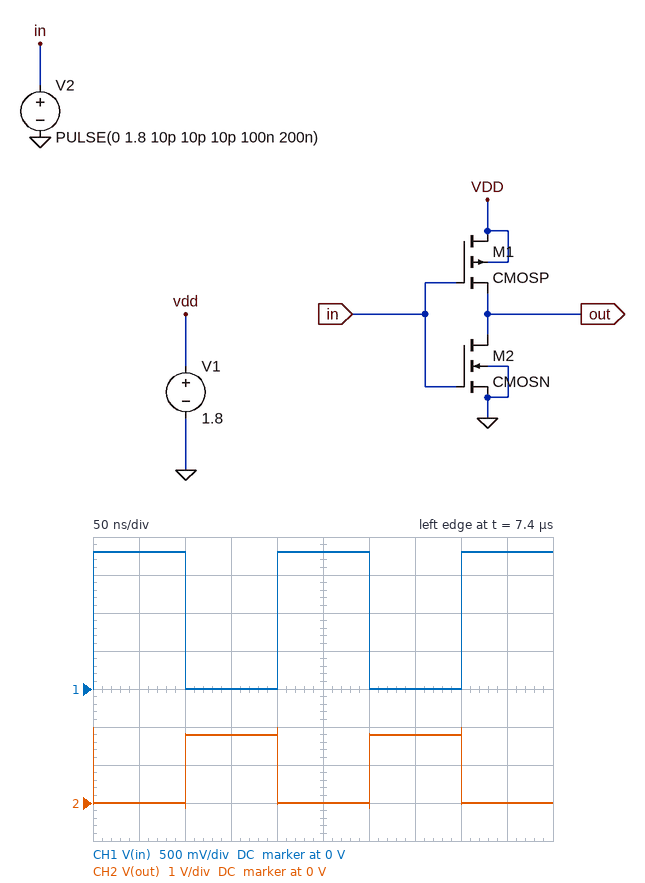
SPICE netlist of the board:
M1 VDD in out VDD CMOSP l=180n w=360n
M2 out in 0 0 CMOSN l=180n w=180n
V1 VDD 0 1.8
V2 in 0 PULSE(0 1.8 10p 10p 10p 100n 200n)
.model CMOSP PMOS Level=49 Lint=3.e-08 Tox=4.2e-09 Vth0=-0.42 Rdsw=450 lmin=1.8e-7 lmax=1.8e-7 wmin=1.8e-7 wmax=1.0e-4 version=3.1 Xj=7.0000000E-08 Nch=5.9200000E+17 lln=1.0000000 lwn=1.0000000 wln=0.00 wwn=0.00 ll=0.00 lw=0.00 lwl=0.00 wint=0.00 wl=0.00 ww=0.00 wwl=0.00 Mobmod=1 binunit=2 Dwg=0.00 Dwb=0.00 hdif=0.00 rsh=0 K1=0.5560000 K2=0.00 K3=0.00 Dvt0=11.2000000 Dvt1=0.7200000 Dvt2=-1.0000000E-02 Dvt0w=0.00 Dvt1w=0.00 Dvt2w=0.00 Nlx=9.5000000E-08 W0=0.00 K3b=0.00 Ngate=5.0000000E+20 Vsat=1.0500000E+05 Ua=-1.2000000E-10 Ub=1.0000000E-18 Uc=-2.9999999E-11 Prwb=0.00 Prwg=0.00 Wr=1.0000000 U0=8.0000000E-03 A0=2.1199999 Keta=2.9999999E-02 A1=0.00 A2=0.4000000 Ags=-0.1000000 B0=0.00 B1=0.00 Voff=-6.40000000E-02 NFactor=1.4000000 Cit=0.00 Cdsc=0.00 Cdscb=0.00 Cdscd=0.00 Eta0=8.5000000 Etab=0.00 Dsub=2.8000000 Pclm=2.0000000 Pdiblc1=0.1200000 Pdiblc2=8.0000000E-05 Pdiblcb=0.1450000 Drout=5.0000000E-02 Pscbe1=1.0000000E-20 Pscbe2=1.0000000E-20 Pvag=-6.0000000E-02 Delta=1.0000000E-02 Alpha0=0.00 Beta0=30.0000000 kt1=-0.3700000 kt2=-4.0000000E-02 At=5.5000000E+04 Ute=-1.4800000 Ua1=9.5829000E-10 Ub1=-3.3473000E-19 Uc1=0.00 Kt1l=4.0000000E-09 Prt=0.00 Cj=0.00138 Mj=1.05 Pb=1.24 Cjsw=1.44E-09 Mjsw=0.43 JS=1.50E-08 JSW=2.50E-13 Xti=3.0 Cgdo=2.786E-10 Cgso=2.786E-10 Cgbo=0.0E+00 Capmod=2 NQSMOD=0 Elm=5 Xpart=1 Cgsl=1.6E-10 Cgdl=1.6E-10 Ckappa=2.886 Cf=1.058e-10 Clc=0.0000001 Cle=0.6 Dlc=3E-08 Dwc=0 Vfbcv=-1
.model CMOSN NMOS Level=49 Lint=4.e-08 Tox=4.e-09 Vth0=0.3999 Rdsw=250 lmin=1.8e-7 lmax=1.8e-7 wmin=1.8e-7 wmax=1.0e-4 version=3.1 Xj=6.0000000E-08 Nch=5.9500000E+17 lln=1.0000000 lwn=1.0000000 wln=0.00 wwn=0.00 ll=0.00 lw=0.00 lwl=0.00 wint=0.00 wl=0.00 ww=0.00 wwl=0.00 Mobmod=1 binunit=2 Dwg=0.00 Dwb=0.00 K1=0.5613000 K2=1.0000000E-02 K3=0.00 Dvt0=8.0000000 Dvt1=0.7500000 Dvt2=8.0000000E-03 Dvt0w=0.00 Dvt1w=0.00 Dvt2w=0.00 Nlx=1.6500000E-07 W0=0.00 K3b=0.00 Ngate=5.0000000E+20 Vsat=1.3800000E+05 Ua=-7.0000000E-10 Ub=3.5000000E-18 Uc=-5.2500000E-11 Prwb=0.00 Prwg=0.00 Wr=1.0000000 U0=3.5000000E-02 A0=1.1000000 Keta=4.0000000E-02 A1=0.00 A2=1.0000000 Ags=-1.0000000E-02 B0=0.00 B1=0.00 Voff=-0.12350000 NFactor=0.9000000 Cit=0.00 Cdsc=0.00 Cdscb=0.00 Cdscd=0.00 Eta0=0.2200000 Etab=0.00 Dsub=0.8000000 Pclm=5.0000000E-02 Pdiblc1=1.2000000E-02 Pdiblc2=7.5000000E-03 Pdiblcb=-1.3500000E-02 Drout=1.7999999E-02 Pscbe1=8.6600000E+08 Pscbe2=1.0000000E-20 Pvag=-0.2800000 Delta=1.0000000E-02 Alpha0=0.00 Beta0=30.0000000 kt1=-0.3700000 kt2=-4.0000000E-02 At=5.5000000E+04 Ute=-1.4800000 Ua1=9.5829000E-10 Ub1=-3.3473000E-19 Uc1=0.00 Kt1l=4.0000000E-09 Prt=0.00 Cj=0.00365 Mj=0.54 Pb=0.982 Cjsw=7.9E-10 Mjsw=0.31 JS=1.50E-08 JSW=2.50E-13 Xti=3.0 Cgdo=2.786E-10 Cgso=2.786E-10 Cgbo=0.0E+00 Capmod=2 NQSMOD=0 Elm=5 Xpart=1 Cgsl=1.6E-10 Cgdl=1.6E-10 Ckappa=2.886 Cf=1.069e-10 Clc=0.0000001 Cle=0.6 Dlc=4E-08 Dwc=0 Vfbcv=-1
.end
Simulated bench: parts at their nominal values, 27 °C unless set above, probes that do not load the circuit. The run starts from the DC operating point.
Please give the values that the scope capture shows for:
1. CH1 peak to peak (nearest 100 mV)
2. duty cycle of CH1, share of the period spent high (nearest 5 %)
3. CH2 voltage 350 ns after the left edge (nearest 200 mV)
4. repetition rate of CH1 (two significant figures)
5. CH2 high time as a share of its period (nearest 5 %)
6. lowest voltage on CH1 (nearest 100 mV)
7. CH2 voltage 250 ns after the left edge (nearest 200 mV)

1.8 V
50 %
1.8 V
5.0 MHz
50 %
0 V
0 V
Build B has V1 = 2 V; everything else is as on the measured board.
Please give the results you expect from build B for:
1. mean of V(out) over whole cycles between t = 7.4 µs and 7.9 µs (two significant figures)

1.0 V
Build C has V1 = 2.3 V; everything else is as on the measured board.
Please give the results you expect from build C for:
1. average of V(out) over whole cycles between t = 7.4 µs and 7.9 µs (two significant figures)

1.2 V
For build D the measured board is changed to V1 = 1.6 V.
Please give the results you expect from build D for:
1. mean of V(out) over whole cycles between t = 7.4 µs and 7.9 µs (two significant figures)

800 mV
